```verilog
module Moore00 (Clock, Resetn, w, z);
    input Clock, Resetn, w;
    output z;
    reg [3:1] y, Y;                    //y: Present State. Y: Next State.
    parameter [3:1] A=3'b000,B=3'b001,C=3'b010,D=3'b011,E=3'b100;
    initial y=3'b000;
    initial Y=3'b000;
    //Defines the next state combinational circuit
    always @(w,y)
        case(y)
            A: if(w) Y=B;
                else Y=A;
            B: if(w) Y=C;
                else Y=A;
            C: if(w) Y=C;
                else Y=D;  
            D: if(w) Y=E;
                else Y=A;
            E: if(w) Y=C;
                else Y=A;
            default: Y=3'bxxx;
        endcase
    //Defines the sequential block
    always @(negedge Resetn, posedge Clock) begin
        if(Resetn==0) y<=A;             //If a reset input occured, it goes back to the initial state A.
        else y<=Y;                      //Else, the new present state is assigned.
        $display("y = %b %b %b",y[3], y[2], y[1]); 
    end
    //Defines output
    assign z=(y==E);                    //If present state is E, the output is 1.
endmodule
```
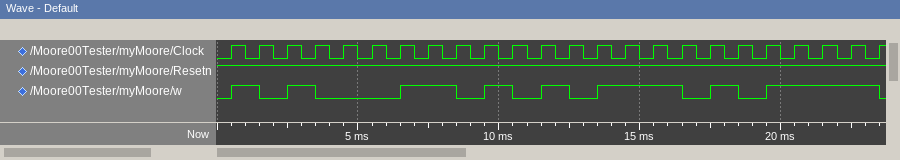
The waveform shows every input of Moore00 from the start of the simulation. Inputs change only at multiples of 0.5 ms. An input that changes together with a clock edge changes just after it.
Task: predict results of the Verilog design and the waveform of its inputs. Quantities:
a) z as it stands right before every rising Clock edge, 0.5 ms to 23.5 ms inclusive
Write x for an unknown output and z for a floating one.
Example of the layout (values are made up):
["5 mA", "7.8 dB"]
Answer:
["0 0 0 0 0 0 0 0 0 0 0 1 0 0 0 0 0 0 0 1 0 0 0 0"]
